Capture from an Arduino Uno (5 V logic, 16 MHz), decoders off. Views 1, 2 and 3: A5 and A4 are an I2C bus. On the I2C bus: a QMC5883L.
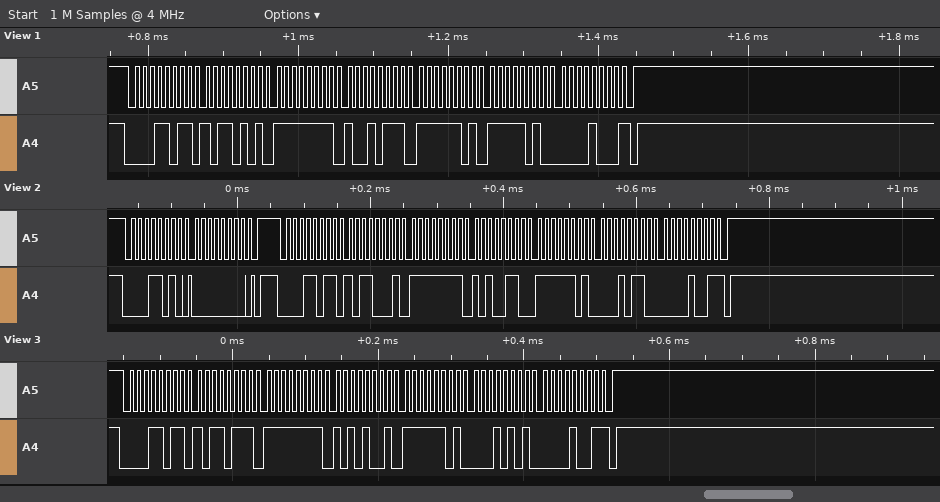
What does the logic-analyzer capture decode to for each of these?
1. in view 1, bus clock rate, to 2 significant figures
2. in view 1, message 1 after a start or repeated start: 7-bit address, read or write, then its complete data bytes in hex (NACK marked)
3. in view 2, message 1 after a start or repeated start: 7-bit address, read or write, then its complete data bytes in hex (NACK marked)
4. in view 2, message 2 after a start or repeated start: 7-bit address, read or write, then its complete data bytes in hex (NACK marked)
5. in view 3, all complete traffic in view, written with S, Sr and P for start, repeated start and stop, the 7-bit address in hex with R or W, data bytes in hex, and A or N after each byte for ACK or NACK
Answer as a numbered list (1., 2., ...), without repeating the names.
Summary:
1. 100 kHz
2. 0x0D read: B5 FF 97 FD FA 08 NACK
3. 0x0D write: 00
4. 0x0D read: B1 FF A6 FD 16 09 NACK
5. S 0DR A B7 A FF A A9 A FD A 15 A 09 N P
